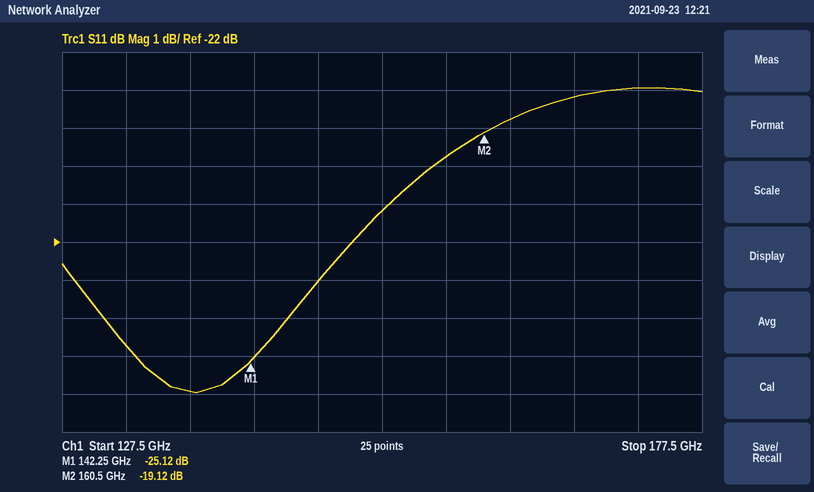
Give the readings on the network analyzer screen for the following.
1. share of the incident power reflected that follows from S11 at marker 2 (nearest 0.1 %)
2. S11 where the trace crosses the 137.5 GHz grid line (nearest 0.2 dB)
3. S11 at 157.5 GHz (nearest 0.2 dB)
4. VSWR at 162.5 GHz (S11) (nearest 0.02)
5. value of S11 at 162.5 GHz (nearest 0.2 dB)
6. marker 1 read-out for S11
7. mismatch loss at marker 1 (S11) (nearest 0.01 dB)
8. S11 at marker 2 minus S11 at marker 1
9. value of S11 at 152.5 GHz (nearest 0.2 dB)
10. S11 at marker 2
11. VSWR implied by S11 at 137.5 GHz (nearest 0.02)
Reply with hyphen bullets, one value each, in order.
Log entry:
- 1.2 %
- -26.0 dB
- -19.8 dB
- 1.26
- -18.8 dB
- -25.12 dB
- 0.01 dB
- 6.00 dB
- -21.2 dB
- -19.12 dB
- 1.10
